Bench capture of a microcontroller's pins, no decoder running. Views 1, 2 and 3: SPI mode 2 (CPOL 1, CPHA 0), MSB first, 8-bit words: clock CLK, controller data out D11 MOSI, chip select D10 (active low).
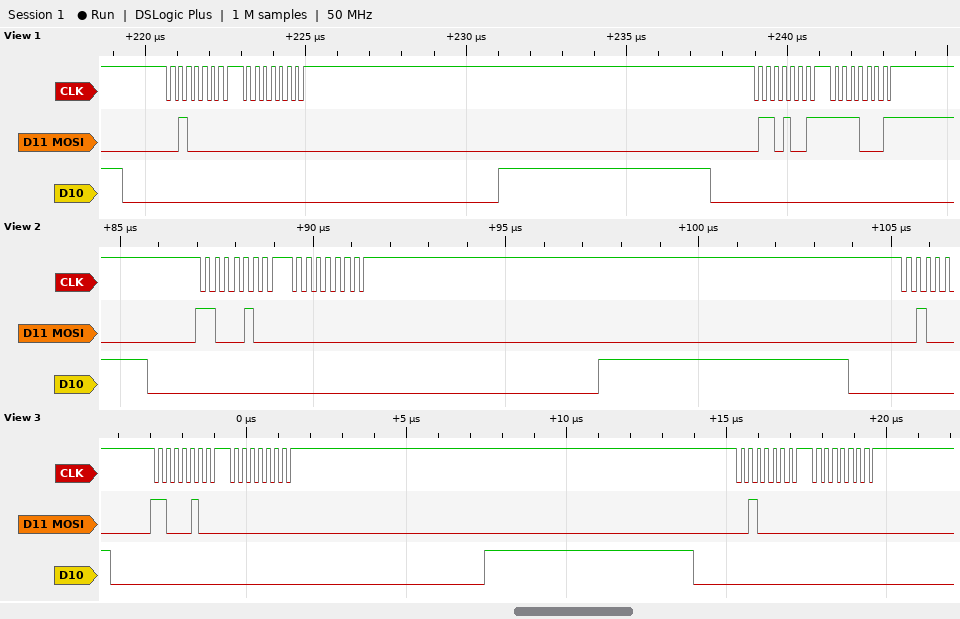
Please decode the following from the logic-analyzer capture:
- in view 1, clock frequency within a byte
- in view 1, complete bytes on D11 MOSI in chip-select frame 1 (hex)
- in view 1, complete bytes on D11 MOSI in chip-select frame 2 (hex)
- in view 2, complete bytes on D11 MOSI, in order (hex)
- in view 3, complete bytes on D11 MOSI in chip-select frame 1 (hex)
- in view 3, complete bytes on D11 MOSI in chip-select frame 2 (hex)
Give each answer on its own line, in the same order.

4 MHz
20 00
69 F1
C4 00
0xC4 0x00
0x20 0x00
